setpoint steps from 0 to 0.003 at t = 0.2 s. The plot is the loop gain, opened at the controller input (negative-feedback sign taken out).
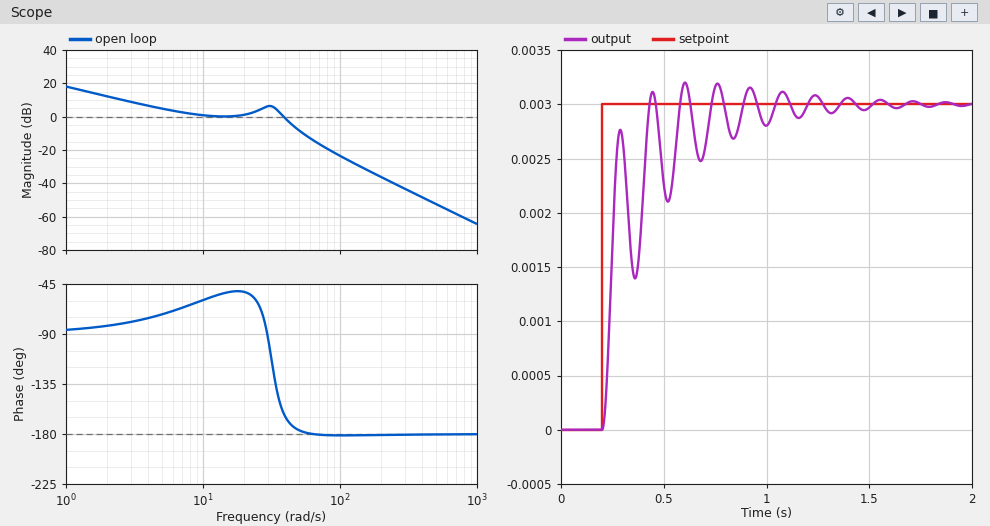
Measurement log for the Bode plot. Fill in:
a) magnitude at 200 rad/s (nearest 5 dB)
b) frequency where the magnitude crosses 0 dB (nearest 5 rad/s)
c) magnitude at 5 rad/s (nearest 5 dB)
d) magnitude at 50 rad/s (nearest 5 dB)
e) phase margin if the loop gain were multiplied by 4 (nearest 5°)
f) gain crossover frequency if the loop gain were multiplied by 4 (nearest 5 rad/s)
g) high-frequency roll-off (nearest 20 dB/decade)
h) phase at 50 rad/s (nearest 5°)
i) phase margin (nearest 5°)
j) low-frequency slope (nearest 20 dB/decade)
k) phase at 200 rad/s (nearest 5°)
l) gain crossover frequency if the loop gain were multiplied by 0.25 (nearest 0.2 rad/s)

-35 dB
40 rad/s
5 dB
-10 dB
0°
60 rad/s
-40 dB/decade
-175°
20°
-20 dB/decade
-180°
2.0 rad/s
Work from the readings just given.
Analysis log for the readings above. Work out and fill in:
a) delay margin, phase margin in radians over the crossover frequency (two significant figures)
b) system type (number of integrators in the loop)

0.0087 s
1
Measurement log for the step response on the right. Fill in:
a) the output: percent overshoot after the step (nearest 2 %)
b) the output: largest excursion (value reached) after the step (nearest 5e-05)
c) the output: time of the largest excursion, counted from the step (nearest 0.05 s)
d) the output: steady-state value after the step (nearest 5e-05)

6 %
0.00320
0.40 s
0.00300
